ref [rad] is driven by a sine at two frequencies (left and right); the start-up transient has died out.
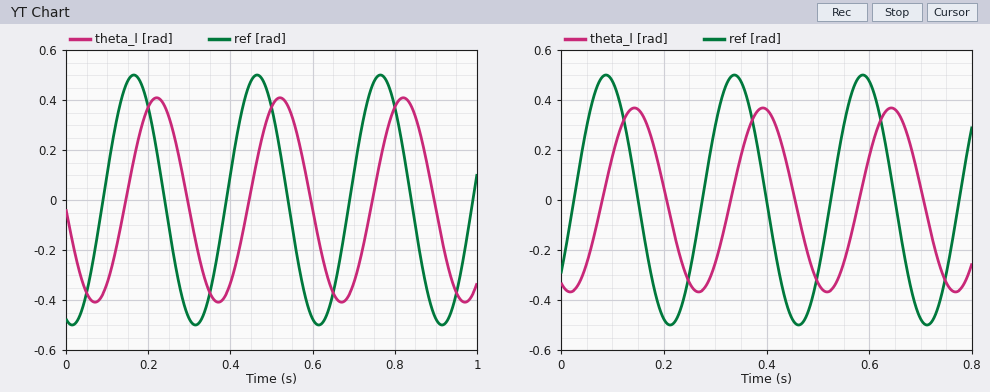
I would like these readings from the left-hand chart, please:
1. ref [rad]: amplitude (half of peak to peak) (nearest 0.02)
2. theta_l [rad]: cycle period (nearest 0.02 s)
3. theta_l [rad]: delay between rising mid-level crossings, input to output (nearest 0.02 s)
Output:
0.50
0.30 s
0.06 s
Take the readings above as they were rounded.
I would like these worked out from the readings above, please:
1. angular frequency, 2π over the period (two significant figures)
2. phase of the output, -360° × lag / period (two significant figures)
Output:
21 rad/s
-72°
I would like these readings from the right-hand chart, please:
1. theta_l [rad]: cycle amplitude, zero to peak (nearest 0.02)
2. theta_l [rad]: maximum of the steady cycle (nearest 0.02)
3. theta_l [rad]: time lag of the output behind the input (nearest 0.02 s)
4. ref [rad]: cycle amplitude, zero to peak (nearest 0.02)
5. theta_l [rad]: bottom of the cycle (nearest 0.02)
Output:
0.36
0.36
0.06 s
0.50
-0.36
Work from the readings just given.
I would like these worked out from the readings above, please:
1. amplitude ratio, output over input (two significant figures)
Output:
0.72
